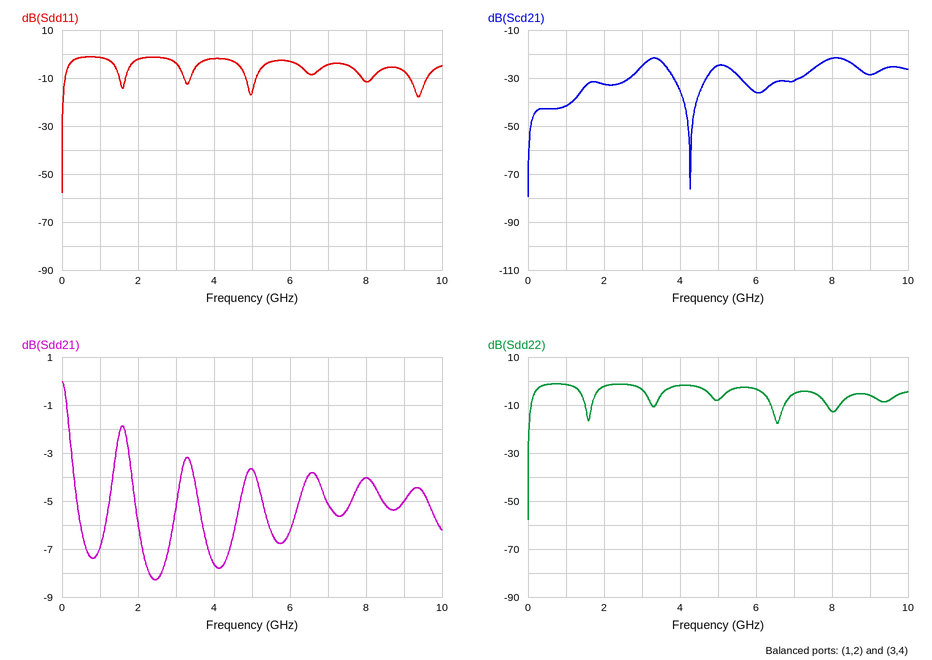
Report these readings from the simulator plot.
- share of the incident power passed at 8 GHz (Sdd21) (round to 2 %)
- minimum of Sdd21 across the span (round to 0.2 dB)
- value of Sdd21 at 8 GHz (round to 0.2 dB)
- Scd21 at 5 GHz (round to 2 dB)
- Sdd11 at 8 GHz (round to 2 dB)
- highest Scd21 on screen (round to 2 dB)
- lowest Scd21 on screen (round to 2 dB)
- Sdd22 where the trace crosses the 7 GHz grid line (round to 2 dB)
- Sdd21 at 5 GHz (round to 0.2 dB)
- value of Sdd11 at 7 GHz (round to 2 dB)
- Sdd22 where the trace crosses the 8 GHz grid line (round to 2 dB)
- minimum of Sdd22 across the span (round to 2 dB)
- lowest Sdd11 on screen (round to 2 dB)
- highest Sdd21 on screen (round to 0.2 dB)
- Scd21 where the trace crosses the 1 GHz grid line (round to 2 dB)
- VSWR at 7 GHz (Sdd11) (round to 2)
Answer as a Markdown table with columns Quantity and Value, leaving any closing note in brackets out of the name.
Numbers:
| Quantity | Value |
|---|---|
| share of the incident power passed at 8 GHz (Sdd21) | 40 % |
| minimum of Sdd21 across the span | -8.2 dB |
| value of Sdd21 at 8 GHz | -4.0 dB |
| Scd21 at 5 GHz | -24 dB |
| Sdd11 at 8 GHz | -12 dB |
| highest Scd21 on screen | -22 dB |
| lowest Scd21 on screen | -80 dB |
| Sdd22 where the trace crosses the 7 GHz grid line | -6 dB |
| Sdd21 at 5 GHz | -3.6 dB |
| value of Sdd11 at 7 GHz | -4 dB |
| Sdd22 where the trace crosses the 8 GHz grid line | -12 dB |
| minimum of Sdd22 across the span | -58 dB |
| lowest Sdd11 on screen | -58 dB |
| highest Sdd21 on screen | 0.0 dB |
| Scd21 where the trace crosses the 1 GHz grid line | -42 dB |
| VSWR at 7 GHz (Sdd11) | 4 |
